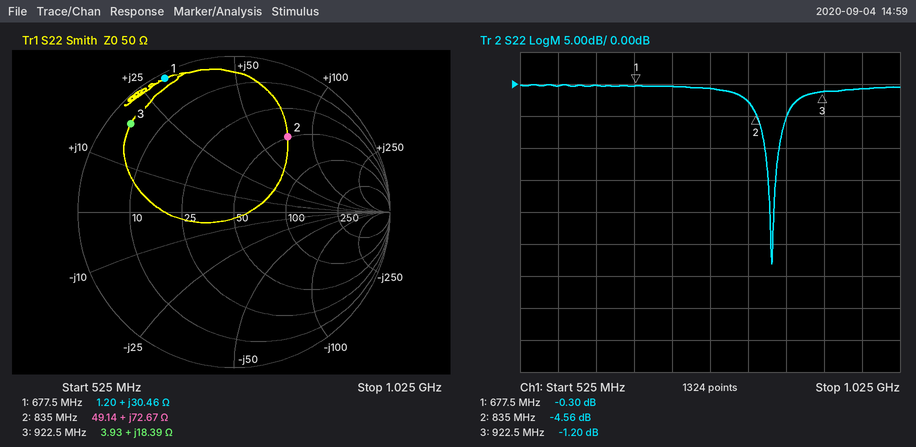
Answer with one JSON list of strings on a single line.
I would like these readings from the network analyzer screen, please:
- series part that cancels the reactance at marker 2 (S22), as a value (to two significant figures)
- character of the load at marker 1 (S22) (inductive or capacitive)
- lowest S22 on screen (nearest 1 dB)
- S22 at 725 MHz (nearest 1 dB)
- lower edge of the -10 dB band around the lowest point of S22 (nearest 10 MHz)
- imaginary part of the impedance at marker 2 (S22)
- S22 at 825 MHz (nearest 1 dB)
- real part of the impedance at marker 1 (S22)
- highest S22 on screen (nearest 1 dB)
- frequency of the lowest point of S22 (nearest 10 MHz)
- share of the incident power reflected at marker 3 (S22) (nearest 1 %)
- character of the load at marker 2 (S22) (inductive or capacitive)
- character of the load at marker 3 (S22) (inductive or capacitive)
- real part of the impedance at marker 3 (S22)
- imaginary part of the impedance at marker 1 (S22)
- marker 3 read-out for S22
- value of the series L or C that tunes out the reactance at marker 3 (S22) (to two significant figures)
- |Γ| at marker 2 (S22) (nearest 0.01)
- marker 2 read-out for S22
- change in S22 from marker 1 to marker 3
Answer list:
["2.6 pF", "inductive", "-28 dB", "0 dB", "850 MHz", "+72.67 Ω", "-3 dB", "1.20 Ω", "0 dB", "860 MHz", "76 %", "inductive", "inductive", "3.93 Ω", "+30.46 Ω", "-1.20 dB", "9.4 pF", "0.59", "-4.56 dB", "-0.90 dB"]
